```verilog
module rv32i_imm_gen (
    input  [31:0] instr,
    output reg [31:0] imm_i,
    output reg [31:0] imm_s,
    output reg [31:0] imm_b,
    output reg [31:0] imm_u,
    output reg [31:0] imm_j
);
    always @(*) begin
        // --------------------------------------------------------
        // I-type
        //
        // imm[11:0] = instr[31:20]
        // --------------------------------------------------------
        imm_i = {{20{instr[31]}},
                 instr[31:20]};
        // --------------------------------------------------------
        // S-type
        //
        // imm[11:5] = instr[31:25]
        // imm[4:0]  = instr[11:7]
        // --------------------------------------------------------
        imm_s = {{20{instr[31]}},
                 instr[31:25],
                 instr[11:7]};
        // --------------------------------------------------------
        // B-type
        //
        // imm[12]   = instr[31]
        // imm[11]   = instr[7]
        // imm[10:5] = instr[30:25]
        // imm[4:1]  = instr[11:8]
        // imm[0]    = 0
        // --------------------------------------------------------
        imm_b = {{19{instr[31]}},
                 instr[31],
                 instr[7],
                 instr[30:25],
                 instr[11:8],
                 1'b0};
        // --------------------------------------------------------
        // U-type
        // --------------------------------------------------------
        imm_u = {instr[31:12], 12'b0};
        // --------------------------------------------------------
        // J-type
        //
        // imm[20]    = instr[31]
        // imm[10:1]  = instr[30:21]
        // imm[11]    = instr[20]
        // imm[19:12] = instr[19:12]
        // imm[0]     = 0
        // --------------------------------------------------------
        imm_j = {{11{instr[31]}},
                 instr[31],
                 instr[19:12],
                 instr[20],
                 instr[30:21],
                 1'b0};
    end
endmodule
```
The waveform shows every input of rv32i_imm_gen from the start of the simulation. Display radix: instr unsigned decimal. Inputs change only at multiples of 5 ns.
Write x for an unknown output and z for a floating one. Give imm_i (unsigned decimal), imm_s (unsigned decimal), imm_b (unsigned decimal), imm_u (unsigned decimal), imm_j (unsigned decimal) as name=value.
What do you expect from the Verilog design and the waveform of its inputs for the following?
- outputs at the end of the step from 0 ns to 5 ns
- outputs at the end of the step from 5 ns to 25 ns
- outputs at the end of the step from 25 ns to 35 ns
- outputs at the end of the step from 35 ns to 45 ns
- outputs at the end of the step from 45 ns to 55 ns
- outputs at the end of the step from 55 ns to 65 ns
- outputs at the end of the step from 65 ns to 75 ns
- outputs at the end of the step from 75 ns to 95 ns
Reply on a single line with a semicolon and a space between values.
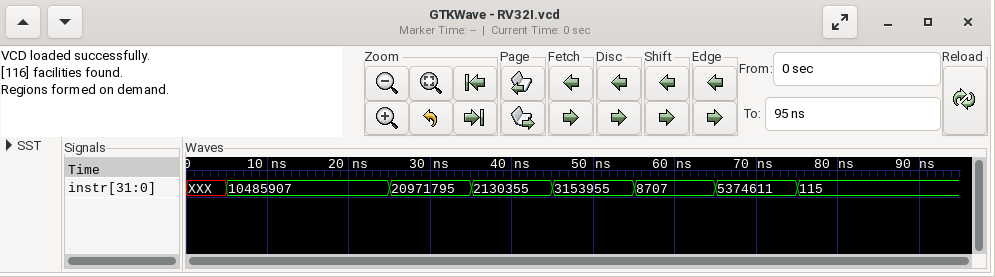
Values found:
imm_i=x, imm_s=x, imm_b=x, imm_u=x, imm_j=x; imm_i=10, imm_s=1, imm_b=2048, imm_u=10485760, imm_j=10; imm_i=20, imm_s=2, imm_b=2, imm_u=20971520, imm_j=20; imm_i=2, imm_s=3, imm_b=2050, imm_u=2129920, imm_j=32770; imm_i=3, imm_s=0, imm_b=0, imm_u=3153920, imm_j=10242; imm_i=0, imm_s=4, imm_b=4, imm_u=8192, imm_j=8192; imm_i=5, imm_s=5, imm_b=2052, imm_u=5373952, imm_j=133124; imm_i=0, imm_s=0, imm_b=0, imm_u=0, imm_j=0
